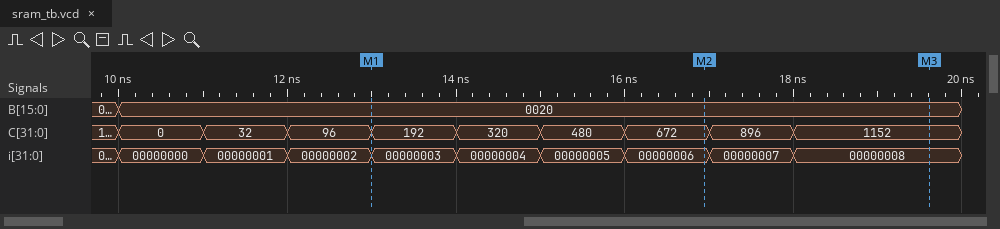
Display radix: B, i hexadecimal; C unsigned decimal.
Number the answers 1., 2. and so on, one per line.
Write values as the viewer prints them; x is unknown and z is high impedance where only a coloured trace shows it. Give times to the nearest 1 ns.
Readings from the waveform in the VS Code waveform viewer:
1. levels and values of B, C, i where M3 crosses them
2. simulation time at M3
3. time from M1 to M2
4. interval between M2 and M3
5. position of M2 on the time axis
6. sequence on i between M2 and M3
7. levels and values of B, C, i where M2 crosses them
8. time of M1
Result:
1. B=0020, C=1152, i=00000008
2. 20 ns
3. 4 ns
4. 3 ns
5. 17 ns
6. 00000006, 00000007, 00000008
7. B=0020, C=672, i=00000006
8. 13 ns
